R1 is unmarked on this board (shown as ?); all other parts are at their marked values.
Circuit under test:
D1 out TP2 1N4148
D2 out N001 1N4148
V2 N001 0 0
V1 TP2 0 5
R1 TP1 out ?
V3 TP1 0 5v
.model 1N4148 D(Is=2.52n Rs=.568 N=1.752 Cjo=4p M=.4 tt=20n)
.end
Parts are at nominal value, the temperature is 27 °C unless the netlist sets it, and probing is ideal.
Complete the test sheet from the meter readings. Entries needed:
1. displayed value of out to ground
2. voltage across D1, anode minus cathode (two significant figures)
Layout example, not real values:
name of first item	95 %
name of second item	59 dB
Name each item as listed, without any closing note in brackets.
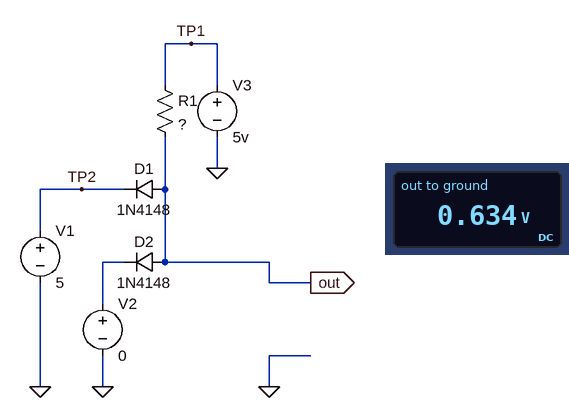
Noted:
displayed value of out to ground	0.634 V
voltage across D1, anode minus cathode	-4.4 V
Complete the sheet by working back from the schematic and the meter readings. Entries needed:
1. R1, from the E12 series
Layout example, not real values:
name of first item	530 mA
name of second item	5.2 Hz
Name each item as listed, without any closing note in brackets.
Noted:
R1, from the E12 series	1.5 kΩ
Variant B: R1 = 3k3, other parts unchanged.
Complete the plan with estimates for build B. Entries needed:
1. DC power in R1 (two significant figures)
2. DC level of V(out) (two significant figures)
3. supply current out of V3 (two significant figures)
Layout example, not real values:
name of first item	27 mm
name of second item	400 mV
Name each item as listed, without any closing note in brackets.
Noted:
DC power in R1	5.9 mW
DC level of V(out)	600 mV
supply current out of V3	1.3 mA
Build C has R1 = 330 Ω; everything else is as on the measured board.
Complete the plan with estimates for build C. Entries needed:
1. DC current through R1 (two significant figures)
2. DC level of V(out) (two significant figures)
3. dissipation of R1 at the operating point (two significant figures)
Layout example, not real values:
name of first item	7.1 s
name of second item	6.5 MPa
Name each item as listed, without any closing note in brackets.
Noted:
DC current through R1	13 mA
DC level of V(out)	710 mV
dissipation of R1 at the operating point	56 mW
